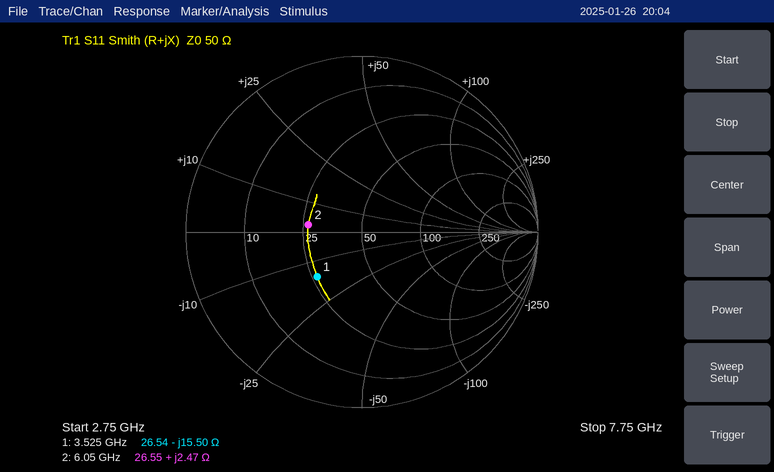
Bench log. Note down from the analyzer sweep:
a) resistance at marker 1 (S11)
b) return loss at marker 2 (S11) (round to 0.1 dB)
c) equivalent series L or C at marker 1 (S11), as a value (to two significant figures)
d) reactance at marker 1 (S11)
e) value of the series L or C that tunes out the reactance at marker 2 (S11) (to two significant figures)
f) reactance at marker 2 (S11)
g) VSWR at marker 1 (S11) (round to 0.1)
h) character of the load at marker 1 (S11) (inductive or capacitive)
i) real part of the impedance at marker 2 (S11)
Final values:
26.54 Ω
10.2 dB
2.9 pF
-15.50 Ω
11 pF
+2.47 Ω
2.1
capacitive
26.55 Ω
